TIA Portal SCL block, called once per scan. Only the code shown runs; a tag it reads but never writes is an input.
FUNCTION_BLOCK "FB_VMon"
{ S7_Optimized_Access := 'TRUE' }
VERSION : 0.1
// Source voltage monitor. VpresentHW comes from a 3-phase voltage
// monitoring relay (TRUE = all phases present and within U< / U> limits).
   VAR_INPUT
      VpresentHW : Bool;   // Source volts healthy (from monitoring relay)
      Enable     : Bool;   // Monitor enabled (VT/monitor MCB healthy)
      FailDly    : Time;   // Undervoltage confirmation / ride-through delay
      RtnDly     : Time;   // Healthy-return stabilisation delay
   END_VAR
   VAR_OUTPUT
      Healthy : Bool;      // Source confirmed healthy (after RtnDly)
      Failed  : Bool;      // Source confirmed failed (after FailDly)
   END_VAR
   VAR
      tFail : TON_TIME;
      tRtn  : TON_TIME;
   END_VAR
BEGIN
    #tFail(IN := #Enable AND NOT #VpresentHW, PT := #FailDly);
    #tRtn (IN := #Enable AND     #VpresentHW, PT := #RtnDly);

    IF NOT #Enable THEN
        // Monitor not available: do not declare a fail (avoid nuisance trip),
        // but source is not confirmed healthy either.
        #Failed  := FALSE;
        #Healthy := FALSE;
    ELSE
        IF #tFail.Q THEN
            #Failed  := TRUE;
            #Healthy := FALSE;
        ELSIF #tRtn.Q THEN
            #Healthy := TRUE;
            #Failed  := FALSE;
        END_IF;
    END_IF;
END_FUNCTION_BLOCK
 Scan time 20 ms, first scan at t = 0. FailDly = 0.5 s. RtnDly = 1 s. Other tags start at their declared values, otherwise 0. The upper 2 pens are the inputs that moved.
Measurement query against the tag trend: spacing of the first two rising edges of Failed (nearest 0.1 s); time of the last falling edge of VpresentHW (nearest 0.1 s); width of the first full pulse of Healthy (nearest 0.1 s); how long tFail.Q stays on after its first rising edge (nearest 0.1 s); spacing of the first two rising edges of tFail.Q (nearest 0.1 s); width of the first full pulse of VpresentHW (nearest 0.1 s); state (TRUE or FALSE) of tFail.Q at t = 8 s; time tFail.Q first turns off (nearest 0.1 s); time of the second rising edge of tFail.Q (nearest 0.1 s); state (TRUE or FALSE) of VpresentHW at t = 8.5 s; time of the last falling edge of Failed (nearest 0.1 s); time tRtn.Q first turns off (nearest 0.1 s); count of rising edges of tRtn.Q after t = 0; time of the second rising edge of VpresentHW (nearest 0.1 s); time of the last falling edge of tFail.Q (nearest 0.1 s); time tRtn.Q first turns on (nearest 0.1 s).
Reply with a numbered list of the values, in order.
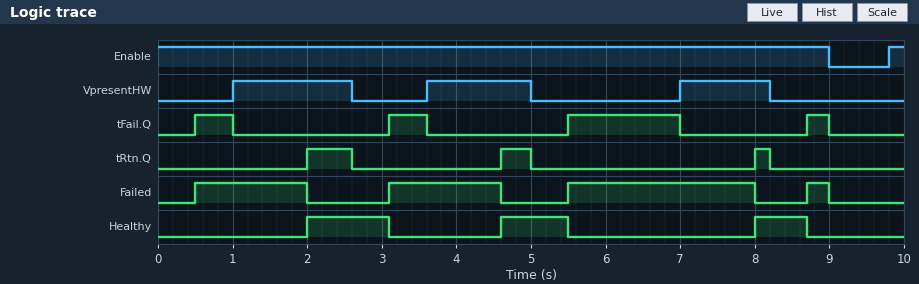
1. 2.6 s
2. 8.2 s
3. 1.1 s
4. 0.5 s
5. 2.6 s
6. 1.6 s
7. FALSE
8. 1.0 s
9. 3.1 s
10. FALSE
11. 9.0 s
12. 2.6 s
13. 3
14. 3.6 s
15. 9.0 s
16. 2.0 s
